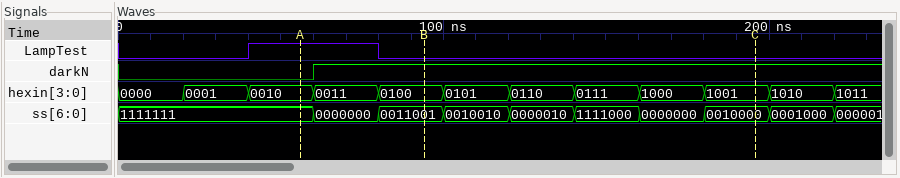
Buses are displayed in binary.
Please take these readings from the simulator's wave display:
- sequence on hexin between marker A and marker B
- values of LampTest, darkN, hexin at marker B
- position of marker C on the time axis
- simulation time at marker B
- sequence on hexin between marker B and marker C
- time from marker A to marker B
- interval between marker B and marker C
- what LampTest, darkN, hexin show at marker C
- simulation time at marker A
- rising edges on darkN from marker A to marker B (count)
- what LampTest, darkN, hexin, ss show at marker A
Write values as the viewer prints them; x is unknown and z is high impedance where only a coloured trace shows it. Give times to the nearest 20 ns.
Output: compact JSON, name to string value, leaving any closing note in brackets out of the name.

{"sequence on hexin between marker A and marker B": "0010, 0011, 0100", "values of LampTest, darkN, hexin at marker B": "LampTest=0, darkN=1, hexin=0100", "position of marker C on the time axis": "200 ns", "simulation time at marker B": "100 ns", "sequence on hexin between marker B and marker C": "0100, 0101, 0110, 0111, 1000, 1001", "time from marker A to marker B": "40 ns", "interval between marker B and marker C": "100 ns", "what LampTest, darkN, hexin show at marker C": "LampTest=0, darkN=1, hexin=1001", "simulation time at marker A": "60 ns", "rising edges on darkN from marker A to marker B": "1", "what LampTest, darkN, hexin, ss show at marker A": "LampTest=1, darkN=0, hexin=0010, ss=1111111"}
